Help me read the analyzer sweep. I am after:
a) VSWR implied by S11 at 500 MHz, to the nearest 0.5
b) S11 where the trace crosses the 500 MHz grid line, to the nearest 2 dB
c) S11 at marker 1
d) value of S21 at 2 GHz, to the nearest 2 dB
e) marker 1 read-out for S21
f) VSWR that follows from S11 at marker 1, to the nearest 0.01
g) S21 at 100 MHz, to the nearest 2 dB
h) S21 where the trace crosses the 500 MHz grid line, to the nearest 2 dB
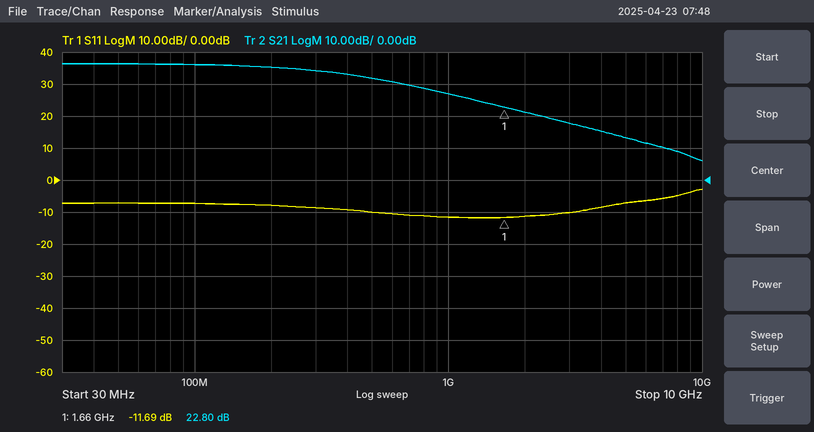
2.0
-10 dB
-11.69 dB
22 dB
22.80 dB
1.70
36 dB
32 dB
